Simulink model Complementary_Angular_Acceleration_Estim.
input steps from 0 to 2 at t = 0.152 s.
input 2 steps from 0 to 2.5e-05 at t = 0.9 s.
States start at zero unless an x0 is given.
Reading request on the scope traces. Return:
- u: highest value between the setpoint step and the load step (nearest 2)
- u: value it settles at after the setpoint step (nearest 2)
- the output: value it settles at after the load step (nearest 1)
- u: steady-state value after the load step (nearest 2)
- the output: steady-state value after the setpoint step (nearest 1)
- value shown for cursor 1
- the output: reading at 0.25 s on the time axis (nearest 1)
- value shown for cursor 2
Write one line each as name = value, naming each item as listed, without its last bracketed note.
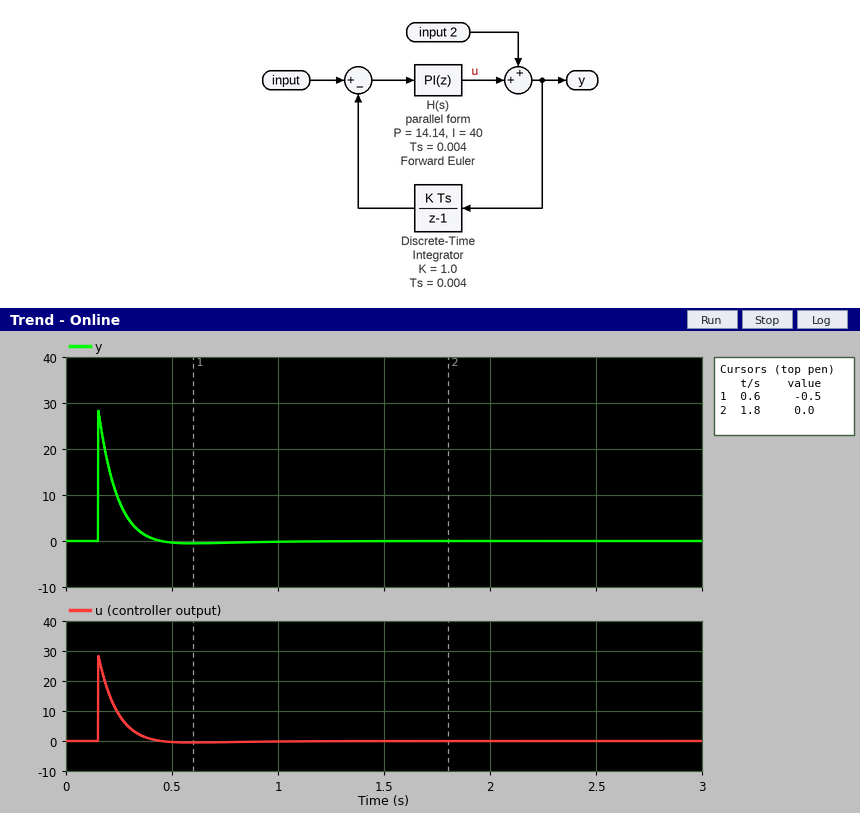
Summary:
u: highest value between the setpoint step and the load step = 28
u: value it settles at after the setpoint step = 0
the output: value it settles at after the load step = 0
u: steady-state value after the load step = 0
the output: steady-state value after the setpoint step = 0
value shown for cursor 1 = -0.5
the output: reading at 0.25 s on the time axis = 9
value shown for cursor 2 = 0.0
